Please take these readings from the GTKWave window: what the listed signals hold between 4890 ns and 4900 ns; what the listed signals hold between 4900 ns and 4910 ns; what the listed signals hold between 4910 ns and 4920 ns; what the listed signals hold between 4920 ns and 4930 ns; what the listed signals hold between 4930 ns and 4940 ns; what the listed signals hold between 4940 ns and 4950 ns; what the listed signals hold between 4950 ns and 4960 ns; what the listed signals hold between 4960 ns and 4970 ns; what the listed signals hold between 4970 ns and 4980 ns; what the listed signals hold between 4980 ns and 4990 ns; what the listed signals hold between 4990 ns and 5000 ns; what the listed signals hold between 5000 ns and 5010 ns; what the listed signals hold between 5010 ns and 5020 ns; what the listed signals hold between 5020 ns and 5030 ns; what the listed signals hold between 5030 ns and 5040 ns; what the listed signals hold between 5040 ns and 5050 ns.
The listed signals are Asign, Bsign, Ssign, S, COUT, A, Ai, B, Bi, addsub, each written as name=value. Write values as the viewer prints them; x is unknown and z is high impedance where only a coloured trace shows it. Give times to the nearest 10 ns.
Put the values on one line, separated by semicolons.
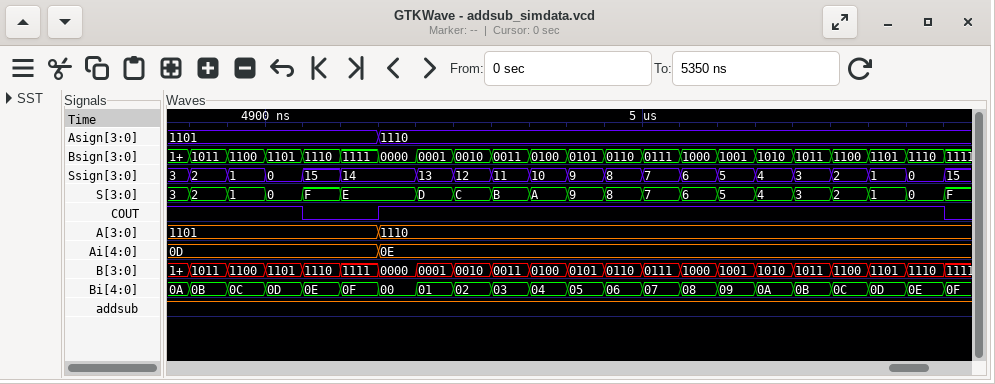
Asign=1101, Bsign=1100, Ssign=1, S=1, COUT=1, A=1101, Ai=0D, B=1100, Bi=0C, addsub=1; Asign=1101, Bsign=1101, Ssign=0, S=0, COUT=1, A=1101, Ai=0D, B=1101, Bi=0D, addsub=1; Asign=1101, Bsign=1110, Ssign=15, S=F, COUT=0, A=1101, Ai=0D, B=1110, Bi=0E, addsub=1; Asign=1101, Bsign=1111, Ssign=14, S=E, COUT=0, A=1101, Ai=0D, B=1111, Bi=0F, addsub=1; Asign=1110, Bsign=0000, Ssign=14, S=E, COUT=1, A=1110, Ai=0E, B=0000, Bi=00, addsub=1; Asign=1110, Bsign=0001, Ssign=13, S=D, COUT=1, A=1110, Ai=0E, B=0001, Bi=01, addsub=1; Asign=1110, Bsign=0010, Ssign=12, S=C, COUT=1, A=1110, Ai=0E, B=0010, Bi=02, addsub=1; Asign=1110, Bsign=0011, Ssign=11, S=B, COUT=1, A=1110, Ai=0E, B=0011, Bi=03, addsub=1; Asign=1110, Bsign=0100, Ssign=10, S=A, COUT=1, A=1110, Ai=0E, B=0100, Bi=04, addsub=1; Asign=1110, Bsign=0101, Ssign=9, S=9, COUT=1, A=1110, Ai=0E, B=0101, Bi=05, addsub=1; Asign=1110, Bsign=0110, Ssign=8, S=8, COUT=1, A=1110, Ai=0E, B=0110, Bi=06, addsub=1; Asign=1110, Bsign=0111, Ssign=7, S=7, COUT=1, A=1110, Ai=0E, B=0111, Bi=07, addsub=1; Asign=1110, Bsign=1000, Ssign=6, S=6, COUT=1, A=1110, Ai=0E, B=1000, Bi=08, addsub=1; Asign=1110, Bsign=1001, Ssign=5, S=5, COUT=1, A=1110, Ai=0E, B=1001, Bi=09, addsub=1; Asign=1110, Bsign=1010, Ssign=4, S=4, COUT=1, A=1110, Ai=0E, B=1010, Bi=0A, addsub=1; Asign=1110, Bsign=1011, Ssign=3, S=3, COUT=1, A=1110, Ai=0E, B=1011, Bi=0B, addsub=1
